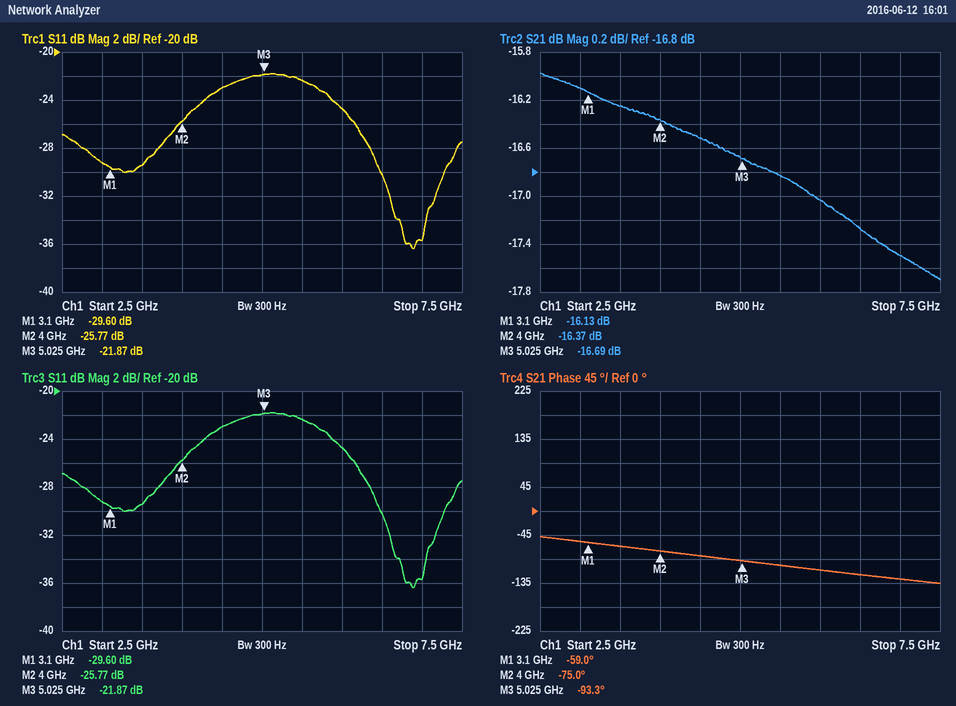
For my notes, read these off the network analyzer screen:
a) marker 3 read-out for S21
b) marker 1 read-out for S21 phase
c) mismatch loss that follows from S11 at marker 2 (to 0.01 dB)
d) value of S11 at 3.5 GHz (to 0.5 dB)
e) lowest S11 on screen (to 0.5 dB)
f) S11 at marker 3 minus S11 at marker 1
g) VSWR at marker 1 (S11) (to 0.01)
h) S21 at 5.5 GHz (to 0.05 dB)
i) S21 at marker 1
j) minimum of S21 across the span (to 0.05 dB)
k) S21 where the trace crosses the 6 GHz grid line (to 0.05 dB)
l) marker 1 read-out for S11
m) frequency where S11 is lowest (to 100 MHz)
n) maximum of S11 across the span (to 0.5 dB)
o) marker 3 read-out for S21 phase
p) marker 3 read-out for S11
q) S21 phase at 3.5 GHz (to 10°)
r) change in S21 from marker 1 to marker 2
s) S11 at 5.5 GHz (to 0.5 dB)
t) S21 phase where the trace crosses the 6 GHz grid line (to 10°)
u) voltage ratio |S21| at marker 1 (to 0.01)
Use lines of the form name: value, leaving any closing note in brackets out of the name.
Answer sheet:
marker 3 read-out for S21: -16.69 dB
marker 1 read-out for S21 phase: -59.0°
mismatch loss that follows from S11 at marker 2: 0.01 dB
value of S11 at 3.5 GHz: -29.5 dB
lowest S11 on screen: -36.5 dB
S11 at marker 3 minus S11 at marker 1: 7.73 dB
VSWR at marker 1 (S11): 1.07
S21 at 5.5 GHz: -16.85 dB
S21 at marker 1: -16.13 dB
minimum of S21 across the span: -17.70 dB
S21 where the trace crosses the 6 GHz grid line: -17.05 dB
marker 1 read-out for S11: -29.60 dB
frequency where S11 is lowest: 6.9 GHz
maximum of S11 across the span: -22.0 dB
marker 3 read-out for S21 phase: -93.3°
marker 3 read-out for S11: -21.87 dB
S21 phase at 3.5 GHz: -70°
change in S21 from marker 1 to marker 2: -0.24 dB
S11 at 5.5 GHz: -22.5 dB
S21 phase where the trace crosses the 6 GHz grid line: -110°
voltage ratio |S21| at marker 1: 0.16
